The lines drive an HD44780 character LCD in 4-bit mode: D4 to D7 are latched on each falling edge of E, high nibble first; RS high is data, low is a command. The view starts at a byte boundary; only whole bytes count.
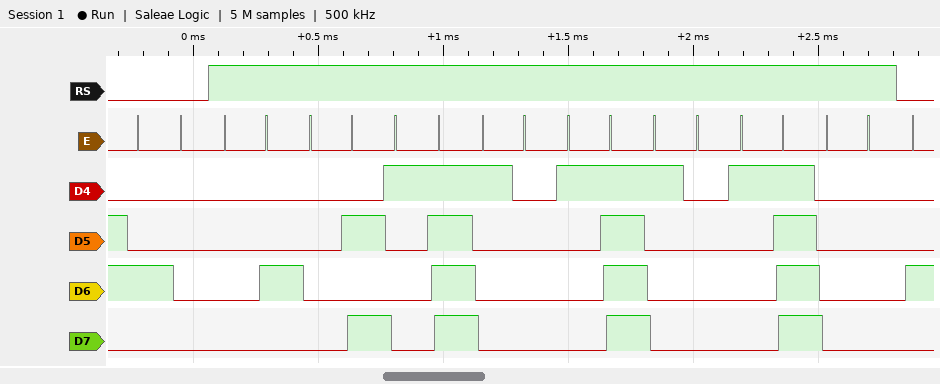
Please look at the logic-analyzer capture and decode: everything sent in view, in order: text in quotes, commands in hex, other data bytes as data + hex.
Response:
0x40 data 04 0A 1F 10 1F 10 1F 00
